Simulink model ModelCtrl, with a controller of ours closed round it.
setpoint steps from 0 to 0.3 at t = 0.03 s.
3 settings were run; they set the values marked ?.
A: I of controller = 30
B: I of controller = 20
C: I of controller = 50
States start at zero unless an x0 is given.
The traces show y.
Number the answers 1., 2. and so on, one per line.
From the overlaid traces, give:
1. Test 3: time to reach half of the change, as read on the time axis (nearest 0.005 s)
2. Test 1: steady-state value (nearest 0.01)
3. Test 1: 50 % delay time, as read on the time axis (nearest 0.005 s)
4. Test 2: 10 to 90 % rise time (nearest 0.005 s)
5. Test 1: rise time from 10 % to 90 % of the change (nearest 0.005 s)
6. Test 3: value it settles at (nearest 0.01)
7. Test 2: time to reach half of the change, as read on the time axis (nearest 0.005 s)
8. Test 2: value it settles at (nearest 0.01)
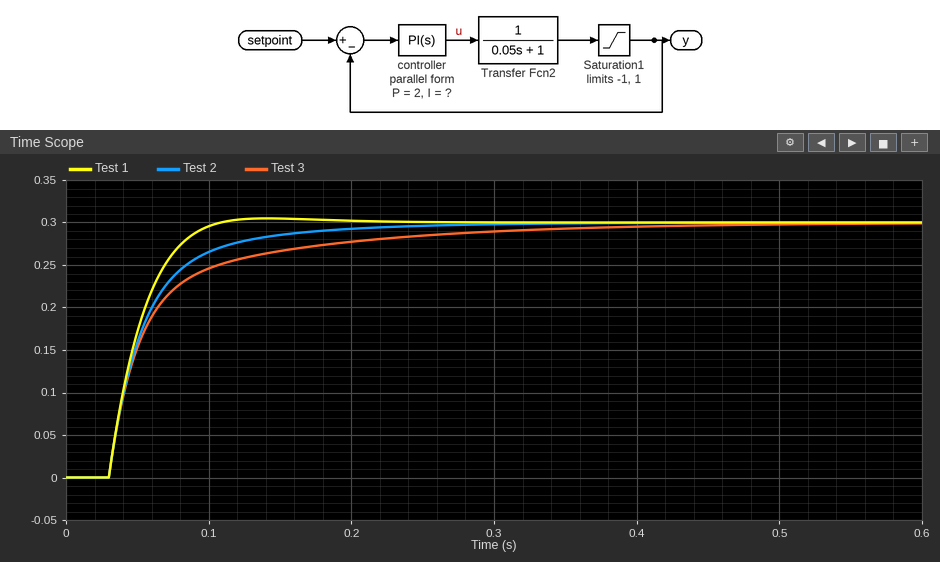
1. 0.050 s
2. 0.30
3. 0.045 s
4. 0.075 s
5. 0.045 s
6. 0.30
7. 0.050 s
8. 0.30
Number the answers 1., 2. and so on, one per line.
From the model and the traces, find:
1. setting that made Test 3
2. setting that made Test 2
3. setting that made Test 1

1. B
2. A
3. C
